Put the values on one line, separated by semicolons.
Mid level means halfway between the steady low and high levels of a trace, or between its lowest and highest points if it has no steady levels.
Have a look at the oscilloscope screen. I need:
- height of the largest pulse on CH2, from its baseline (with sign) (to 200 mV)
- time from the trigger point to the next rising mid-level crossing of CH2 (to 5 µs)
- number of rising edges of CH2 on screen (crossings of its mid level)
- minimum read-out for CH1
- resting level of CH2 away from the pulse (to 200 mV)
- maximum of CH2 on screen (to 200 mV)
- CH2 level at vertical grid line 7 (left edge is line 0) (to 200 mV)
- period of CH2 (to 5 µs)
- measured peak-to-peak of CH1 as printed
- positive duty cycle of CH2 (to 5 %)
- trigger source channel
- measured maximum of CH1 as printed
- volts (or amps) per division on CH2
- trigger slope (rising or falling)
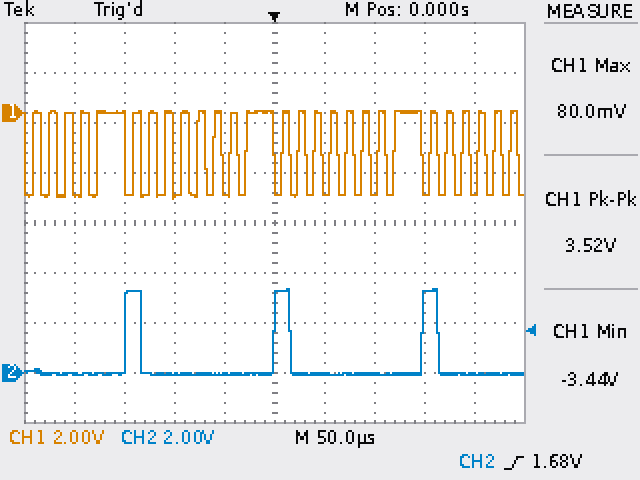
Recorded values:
+3.4 V; 150 µs; 3; -3.44 V; 0.0 V; 3.4 V; 0.0 V; 150 µs; 3.52 V; 10 %; CH2; 80.0 mV; 2 V; rising
